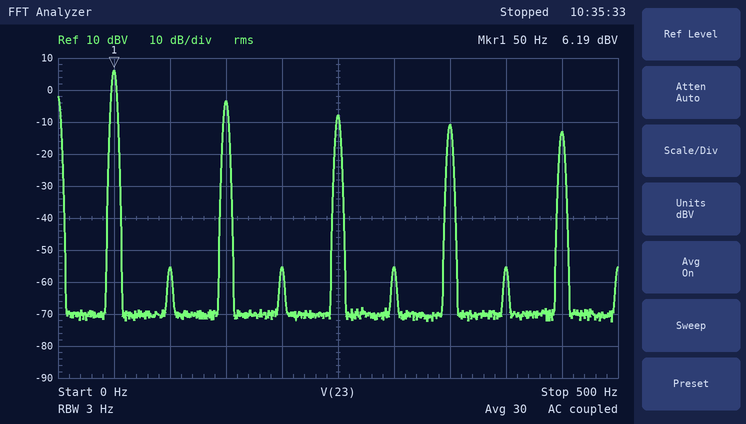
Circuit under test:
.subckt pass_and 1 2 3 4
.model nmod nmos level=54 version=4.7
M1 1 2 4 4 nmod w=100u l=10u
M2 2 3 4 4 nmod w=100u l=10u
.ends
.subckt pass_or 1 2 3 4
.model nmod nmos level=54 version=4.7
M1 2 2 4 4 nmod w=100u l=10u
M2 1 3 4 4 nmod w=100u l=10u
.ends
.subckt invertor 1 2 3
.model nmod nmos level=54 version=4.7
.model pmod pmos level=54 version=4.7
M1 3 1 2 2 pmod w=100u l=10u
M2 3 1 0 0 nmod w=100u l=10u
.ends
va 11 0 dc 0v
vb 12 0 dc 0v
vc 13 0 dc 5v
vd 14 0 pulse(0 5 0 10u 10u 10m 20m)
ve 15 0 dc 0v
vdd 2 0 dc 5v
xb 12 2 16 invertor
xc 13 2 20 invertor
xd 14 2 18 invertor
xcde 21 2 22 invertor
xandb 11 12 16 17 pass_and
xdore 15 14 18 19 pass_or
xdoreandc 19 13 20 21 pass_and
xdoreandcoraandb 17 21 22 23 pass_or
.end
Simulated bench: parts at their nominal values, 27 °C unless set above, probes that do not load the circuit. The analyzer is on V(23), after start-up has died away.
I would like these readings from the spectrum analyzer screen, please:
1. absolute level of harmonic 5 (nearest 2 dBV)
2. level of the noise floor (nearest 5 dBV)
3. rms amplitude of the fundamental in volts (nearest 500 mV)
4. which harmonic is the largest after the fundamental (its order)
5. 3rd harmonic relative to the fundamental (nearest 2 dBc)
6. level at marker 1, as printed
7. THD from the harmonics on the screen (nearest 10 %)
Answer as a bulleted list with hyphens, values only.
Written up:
- -8 dBV
- -70 dBV
- 2.0 V
- 3
- -10 dBc
- 6.19 dBV
- 40 %
